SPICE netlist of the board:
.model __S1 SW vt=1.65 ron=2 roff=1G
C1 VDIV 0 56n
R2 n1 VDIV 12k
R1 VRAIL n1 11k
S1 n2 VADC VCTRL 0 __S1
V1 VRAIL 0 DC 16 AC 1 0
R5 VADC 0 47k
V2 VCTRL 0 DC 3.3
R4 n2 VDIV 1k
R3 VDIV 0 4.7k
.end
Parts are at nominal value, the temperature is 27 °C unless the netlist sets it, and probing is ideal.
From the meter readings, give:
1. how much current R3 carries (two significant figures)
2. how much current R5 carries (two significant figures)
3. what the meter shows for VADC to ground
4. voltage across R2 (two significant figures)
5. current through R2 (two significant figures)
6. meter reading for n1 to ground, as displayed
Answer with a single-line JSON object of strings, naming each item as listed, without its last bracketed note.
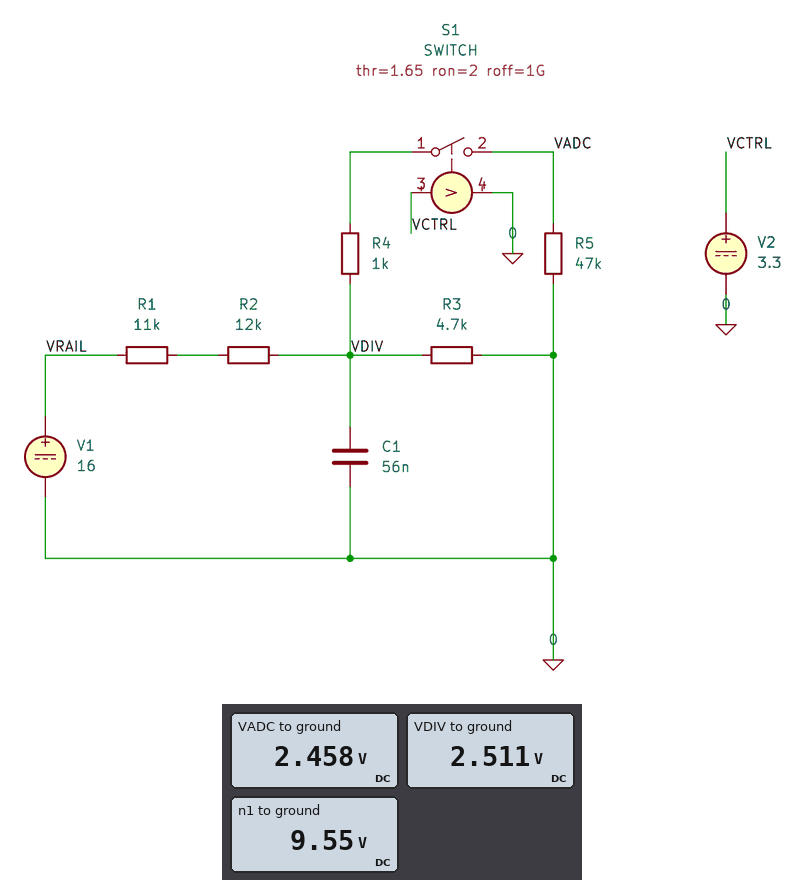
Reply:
{"how much current R3 carries": "530 µA", "how much current R5 carries": "52 µA", "what the meter shows for VADC to ground": "2.458 V", "voltage across R2": "7.0 V", "current through R2": "590 µA", "meter reading for n1 to ground, as displayed": "9.55 V"}
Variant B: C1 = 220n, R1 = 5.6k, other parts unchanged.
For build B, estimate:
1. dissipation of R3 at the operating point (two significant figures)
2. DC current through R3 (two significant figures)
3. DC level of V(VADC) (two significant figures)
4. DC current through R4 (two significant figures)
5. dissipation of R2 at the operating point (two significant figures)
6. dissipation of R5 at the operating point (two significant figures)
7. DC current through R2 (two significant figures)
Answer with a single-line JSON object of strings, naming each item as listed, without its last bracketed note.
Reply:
{"dissipation of R3 at the operating point": "2.1 mW", "DC current through R3": "670 µA", "DC level of V(VADC)": "3.1 V", "DC current through R4": "65 µA", "dissipation of R2 at the operating point": "6.4 mW", "dissipation of R5 at the operating point": "200 µW", "DC current through R2": "730 µA"}
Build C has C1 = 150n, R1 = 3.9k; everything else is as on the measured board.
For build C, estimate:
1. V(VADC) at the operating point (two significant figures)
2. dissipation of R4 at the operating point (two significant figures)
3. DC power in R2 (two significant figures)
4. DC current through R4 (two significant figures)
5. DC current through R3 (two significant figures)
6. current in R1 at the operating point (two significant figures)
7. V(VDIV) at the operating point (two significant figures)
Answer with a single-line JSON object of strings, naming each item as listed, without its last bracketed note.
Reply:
{"V(VADC) at the operating point": "3.3 V", "dissipation of R4 at the operating point": "5.0 µW", "DC power in R2": "7.5 mW", "DC current through R4": "71 µA", "DC current through R3": "720 µA", "current in R1 at the operating point": "790 µA", "V(VDIV) at the operating point": "3.4 V"}
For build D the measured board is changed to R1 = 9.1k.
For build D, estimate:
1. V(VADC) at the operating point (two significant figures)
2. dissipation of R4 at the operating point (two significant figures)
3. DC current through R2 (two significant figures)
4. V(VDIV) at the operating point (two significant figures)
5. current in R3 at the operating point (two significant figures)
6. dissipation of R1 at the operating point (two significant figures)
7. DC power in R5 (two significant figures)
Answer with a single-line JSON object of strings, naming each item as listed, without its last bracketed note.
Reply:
{"V(VADC) at the operating point": "2.6 V", "dissipation of R4 at the operating point": "3.2 µW", "DC current through R2": "630 µA", "V(VDIV) at the operating point": "2.7 V", "current in R3 at the operating point": "570 µA", "dissipation of R1 at the operating point": "3.6 mW", "DC power in R5": "150 µW"}
